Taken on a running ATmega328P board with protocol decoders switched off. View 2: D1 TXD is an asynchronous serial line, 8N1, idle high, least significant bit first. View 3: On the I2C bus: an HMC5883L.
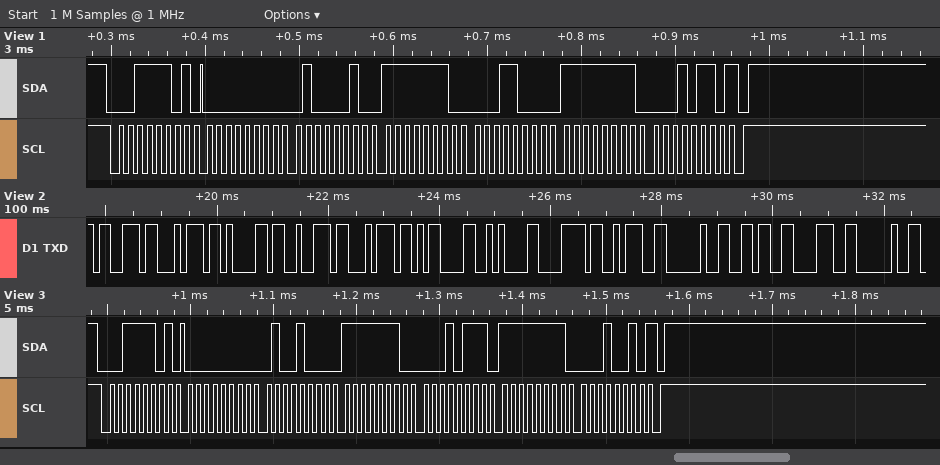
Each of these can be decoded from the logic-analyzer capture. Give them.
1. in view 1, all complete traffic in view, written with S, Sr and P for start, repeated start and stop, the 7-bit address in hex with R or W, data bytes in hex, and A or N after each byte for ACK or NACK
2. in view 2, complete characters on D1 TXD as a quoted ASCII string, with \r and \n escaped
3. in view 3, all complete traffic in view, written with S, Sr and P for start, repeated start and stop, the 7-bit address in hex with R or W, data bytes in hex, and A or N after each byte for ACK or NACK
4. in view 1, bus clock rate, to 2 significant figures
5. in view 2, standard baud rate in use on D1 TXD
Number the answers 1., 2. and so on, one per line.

1. S 1ER A 00 A 42 A FE A 18 A FF A 16 N P
2. "start\r\nx: 68 "
3. S 1ER A 00 A 48 A FE A 17 A FF A 12 N P
4. 100 kHz
5. 9600 baud
